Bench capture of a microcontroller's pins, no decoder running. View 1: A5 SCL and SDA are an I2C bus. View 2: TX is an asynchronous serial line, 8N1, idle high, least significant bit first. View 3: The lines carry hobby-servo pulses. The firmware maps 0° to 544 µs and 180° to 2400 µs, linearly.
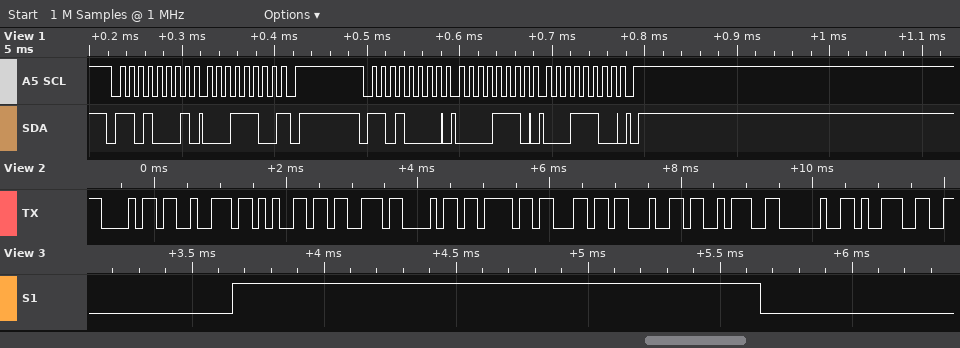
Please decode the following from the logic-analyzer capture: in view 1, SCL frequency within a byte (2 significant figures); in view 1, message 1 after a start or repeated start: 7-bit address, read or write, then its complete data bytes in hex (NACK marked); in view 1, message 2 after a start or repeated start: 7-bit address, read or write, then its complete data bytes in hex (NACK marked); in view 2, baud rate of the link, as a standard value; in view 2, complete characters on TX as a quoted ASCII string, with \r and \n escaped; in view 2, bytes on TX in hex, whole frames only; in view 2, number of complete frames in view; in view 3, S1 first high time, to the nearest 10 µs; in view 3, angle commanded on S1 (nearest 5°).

100 kHz
0x68 read: 1C NACK
0x68 write: 0E 1C
9600 baud
"hreshold: 9"
68 72 65 73 68 6F 6C 64 3A 20 39
11
2000 µs
140°
